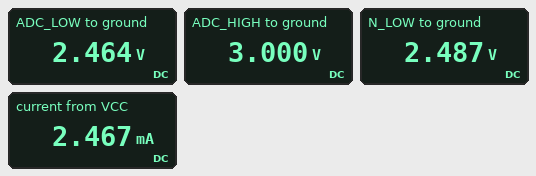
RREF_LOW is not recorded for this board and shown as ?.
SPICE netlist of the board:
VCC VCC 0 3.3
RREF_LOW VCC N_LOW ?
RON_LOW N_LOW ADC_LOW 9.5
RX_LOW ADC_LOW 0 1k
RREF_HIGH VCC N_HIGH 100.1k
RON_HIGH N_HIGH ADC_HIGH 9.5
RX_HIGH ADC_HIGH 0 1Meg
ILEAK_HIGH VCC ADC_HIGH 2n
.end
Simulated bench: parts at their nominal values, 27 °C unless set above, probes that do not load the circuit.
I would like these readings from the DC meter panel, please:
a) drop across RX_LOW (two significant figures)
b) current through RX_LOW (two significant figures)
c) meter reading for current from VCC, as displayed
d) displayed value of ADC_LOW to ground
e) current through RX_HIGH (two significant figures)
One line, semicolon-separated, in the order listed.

2.5 V; 2.5 mA; 2.467 mA; 2.464 V; 3.0 µA
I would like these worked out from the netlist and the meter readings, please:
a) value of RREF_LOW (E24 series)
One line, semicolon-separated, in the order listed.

330 Ω
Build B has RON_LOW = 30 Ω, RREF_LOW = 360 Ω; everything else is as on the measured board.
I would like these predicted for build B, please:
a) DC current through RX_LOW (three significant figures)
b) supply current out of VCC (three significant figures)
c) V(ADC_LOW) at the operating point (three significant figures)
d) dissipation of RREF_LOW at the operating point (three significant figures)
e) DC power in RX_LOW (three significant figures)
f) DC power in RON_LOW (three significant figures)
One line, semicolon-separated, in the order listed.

2.37 mA; 2.38 mA; 2.37 V; 2.03 mW; 5.64 mW; 169 µW
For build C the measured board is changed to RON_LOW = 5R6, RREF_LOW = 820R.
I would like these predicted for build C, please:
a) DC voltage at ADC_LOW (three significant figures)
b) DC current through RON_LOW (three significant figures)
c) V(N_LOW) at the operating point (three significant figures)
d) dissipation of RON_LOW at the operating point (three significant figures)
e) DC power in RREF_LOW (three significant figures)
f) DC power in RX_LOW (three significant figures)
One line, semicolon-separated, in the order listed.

1.81 V; 1.81 mA; 1.82 V; 18.3 µW; 2.68 mW; 3.27 mW
